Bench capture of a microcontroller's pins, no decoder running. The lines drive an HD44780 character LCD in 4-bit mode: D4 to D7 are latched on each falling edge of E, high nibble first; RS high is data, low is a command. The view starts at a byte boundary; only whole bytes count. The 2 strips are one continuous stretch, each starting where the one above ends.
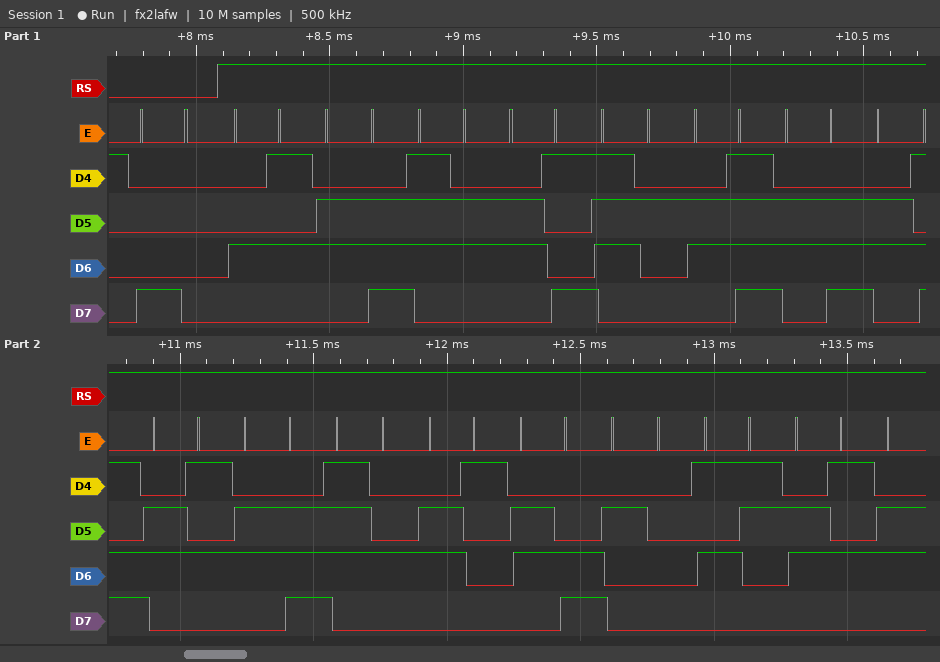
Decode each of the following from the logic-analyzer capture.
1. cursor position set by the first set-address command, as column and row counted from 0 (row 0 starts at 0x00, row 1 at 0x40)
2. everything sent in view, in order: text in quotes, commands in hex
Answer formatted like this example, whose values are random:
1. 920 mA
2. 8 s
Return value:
1. column 0, row 0
2. 0x80 "Environmental Se"
